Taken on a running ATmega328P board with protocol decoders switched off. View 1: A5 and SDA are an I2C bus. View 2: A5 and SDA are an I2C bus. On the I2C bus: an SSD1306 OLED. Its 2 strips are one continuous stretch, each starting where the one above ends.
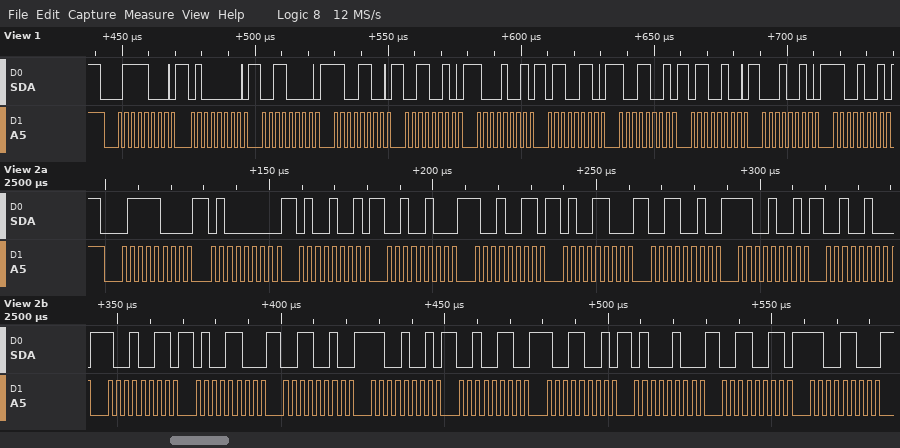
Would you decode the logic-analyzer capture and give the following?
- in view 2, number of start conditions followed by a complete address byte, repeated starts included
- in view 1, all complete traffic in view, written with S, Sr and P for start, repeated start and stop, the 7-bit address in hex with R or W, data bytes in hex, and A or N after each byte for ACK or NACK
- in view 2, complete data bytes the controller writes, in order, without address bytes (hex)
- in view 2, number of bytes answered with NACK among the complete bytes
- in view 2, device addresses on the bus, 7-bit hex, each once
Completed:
1
S 3CW A 40 A 30 A CC A 32 A 89 A 66 A 99 A 64 A 12 A C9 A
40 49 24 93 4C 32 C9 24 93 4C 32 C9 26 99 44 33 CC
0
0x3C
